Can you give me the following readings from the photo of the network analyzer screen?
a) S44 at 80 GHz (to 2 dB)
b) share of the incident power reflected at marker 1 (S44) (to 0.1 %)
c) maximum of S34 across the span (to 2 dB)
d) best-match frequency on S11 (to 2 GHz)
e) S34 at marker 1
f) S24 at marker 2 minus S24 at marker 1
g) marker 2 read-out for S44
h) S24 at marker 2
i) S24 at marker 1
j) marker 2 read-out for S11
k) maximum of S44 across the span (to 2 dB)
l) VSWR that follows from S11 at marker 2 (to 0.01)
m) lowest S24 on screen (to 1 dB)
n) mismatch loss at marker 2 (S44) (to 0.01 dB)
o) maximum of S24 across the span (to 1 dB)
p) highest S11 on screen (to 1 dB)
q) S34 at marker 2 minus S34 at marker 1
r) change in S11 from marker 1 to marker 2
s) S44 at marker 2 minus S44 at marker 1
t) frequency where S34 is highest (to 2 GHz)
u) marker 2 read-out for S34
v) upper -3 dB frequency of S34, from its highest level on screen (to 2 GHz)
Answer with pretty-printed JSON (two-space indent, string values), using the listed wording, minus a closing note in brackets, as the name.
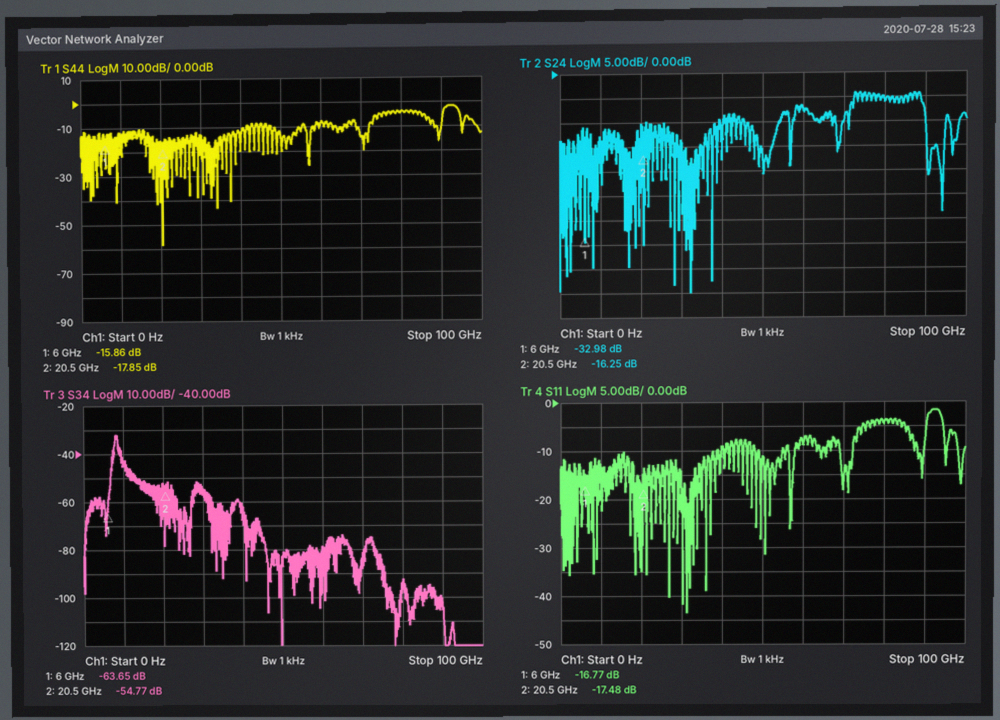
{
  "S44 at 80 GHz": "-4 dB",
  "share of the incident power reflected at marker 1 (S44)": "2.6 %",
  "maximum of S34 across the span": "-32 dB",
  "best-match frequency on S11": "32 GHz",
  "S34 at marker 1": "-63.65 dB",
  "S24 at marker 2 minus S24 at marker 1": "16.73 dB",
  "marker 2 read-out for S44": "-17.85 dB",
  "S24 at marker 2": "-16.25 dB",
  "S24 at marker 1": "-32.98 dB",
  "marker 2 read-out for S11": "-17.48 dB",
  "maximum of S44 across the span": "-2 dB",
  "VSWR that follows from S11 at marker 2": "1.31",
  "lowest S24 on screen": "-45 dB",
  "mismatch loss at marker 2 (S44)": "0.07 dB",
  "maximum of S24 across the span": "-4 dB",
  "highest S11 on screen": "-2 dB",
  "S34 at marker 2 minus S34 at marker 1": "8.88 dB",
  "change in S11 from marker 1 to marker 2": "-0.71 dB",
  "S44 at marker 2 minus S44 at marker 1": "-1.99 dB",
  "frequency where S34 is highest": "8 GHz",
  "marker 2 read-out for S34": "-54.77 dB",
  "upper -3 dB frequency of S34, from its highest level on screen": "8 GHz"
}
